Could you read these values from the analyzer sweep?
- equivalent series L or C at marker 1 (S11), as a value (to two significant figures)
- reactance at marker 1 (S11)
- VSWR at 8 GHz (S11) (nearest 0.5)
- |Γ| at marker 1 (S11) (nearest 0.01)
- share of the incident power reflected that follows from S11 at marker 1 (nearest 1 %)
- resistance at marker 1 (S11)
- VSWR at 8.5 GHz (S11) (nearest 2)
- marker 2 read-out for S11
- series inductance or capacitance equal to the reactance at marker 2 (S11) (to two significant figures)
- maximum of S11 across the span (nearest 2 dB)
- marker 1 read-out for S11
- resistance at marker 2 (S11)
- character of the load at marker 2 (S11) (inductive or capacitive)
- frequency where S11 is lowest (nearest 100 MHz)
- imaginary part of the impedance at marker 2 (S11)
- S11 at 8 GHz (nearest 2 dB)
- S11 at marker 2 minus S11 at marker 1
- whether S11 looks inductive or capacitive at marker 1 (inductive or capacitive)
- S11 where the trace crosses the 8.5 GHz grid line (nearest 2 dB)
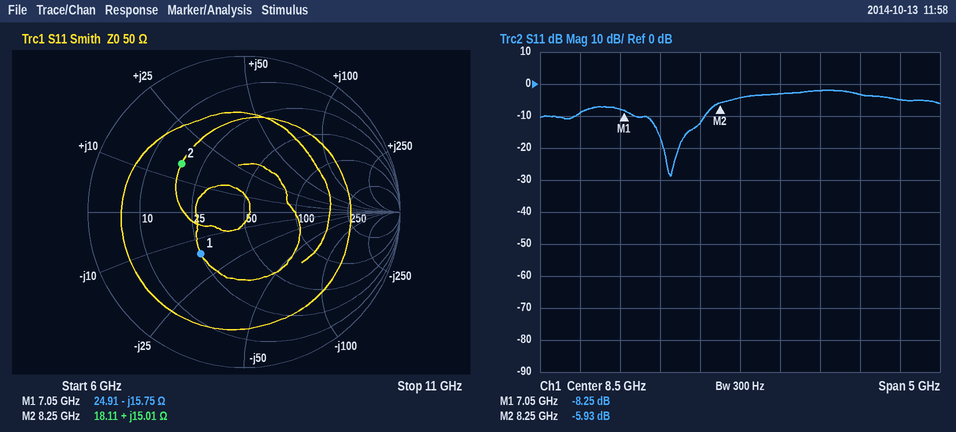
1.4 pF
-15.75 Ω
1.5
0.39
15 %
24.91 Ω
4
-5.93 dB
290 pH
-2 dB
-8.25 dB
18.11 Ω
inductive
7.6 GHz
+15.01 Ω
-12 dB
2.32 dB
capacitive
-4 dB
